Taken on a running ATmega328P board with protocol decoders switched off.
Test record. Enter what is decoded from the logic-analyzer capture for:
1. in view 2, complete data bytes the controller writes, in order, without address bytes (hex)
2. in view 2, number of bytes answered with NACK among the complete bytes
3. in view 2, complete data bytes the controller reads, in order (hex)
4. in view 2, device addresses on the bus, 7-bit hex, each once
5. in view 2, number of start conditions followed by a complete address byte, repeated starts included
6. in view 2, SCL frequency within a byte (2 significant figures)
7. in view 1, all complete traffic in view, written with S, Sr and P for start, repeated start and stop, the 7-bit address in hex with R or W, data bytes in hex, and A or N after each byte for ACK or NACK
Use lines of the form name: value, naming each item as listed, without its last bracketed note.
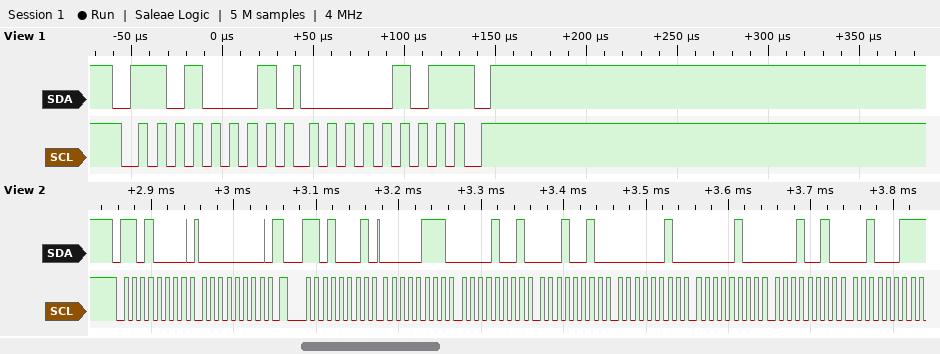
in view 2, complete data bytes the controller writes, in order, without address bytes: 00
in view 2, number of bytes answered with NACK among the complete bytes: 1
in view 2, complete data bytes the controller reads, in order: 07 09 12 02 04 12 23
in view 2, device addresses on the bus, 7-bit hex, each once: 0x68
in view 2, number of start conditions followed by a complete address byte, repeated starts included: 2
in view 2, SCL frequency within a byte: 100 kHz
in view 1, all complete traffic in view, written with S, Sr and P for start, repeated start and stop, the 7-bit address in hex with R or W, data bytes in hex, and A or N after each byte for ACK or NACK: S 68R A 05 N P
